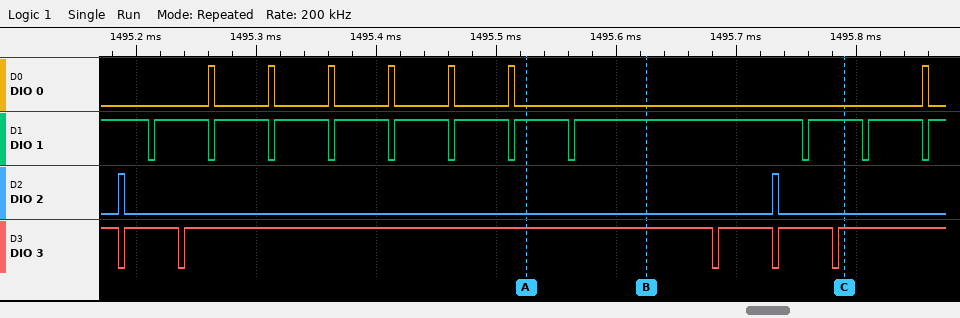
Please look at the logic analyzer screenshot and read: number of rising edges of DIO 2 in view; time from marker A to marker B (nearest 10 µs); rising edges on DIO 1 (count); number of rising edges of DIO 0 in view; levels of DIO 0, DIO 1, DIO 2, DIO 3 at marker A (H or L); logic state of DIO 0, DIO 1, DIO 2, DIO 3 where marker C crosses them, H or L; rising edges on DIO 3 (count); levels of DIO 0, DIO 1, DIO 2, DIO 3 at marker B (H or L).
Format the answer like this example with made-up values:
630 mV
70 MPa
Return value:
2
100 µs
11
7
DIO 0=L, DIO 1=H, DIO 2=L, DIO 3=H
DIO 0=L, DIO 1=H, DIO 2=L, DIO 3=H
5
DIO 0=L, DIO 1=H, DIO 2=L, DIO 3=H
